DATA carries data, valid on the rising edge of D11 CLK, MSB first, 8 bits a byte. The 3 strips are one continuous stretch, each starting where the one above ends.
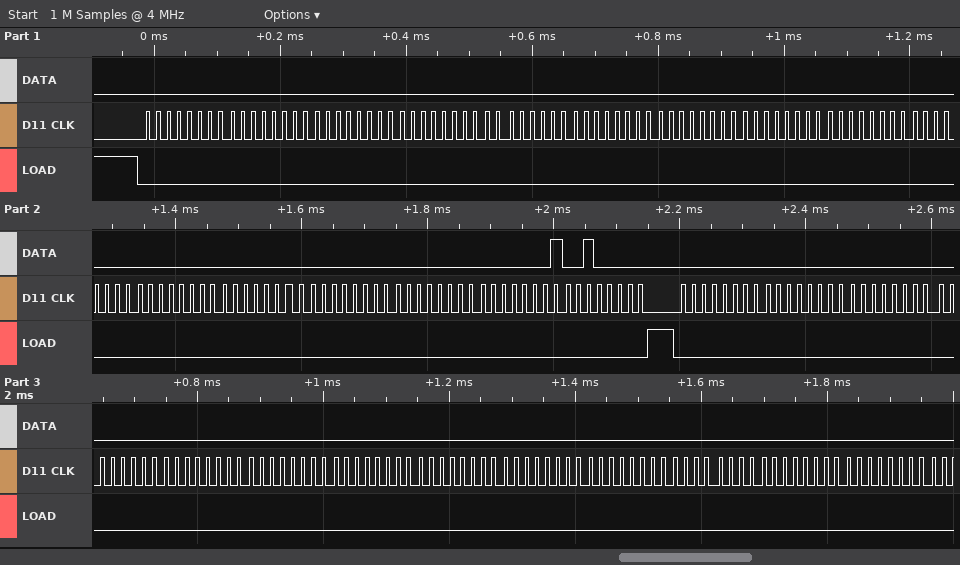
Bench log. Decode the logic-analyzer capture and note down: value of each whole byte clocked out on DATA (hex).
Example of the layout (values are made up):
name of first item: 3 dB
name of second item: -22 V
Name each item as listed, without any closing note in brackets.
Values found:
value of each whole byte clocked out on DATA: 0x00 0x00 0x00 0x00 0x00 0x00 0x00 0x00 0x00 0x00 0x00 0x00 0x00 0x00 0x01 0x20 0x00 0x00 0x00 0x00 0x00 0x00 0x00 0x00 0x00 0x00 0x00 0x00 0x00
